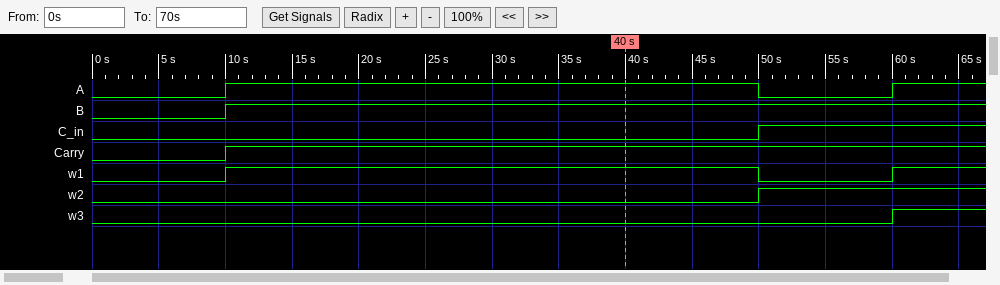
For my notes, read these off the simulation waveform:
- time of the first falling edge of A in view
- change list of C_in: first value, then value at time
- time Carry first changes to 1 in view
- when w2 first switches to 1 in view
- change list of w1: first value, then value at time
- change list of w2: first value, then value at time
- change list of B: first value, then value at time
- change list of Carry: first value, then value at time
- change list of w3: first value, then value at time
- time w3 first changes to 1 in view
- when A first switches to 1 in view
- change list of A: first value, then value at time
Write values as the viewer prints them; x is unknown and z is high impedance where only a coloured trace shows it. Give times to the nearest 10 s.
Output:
50 s
0, 1 at 50 s
10 s
50 s
0, 1 at 10 s, 0 at 50 s, 1 at 60 s
0, 1 at 50 s
0, 1 at 10 s
0, 1 at 10 s
0, 1 at 60 s
60 s
10 s
0, 1 at 10 s, 0 at 50 s, 1 at 60 s
